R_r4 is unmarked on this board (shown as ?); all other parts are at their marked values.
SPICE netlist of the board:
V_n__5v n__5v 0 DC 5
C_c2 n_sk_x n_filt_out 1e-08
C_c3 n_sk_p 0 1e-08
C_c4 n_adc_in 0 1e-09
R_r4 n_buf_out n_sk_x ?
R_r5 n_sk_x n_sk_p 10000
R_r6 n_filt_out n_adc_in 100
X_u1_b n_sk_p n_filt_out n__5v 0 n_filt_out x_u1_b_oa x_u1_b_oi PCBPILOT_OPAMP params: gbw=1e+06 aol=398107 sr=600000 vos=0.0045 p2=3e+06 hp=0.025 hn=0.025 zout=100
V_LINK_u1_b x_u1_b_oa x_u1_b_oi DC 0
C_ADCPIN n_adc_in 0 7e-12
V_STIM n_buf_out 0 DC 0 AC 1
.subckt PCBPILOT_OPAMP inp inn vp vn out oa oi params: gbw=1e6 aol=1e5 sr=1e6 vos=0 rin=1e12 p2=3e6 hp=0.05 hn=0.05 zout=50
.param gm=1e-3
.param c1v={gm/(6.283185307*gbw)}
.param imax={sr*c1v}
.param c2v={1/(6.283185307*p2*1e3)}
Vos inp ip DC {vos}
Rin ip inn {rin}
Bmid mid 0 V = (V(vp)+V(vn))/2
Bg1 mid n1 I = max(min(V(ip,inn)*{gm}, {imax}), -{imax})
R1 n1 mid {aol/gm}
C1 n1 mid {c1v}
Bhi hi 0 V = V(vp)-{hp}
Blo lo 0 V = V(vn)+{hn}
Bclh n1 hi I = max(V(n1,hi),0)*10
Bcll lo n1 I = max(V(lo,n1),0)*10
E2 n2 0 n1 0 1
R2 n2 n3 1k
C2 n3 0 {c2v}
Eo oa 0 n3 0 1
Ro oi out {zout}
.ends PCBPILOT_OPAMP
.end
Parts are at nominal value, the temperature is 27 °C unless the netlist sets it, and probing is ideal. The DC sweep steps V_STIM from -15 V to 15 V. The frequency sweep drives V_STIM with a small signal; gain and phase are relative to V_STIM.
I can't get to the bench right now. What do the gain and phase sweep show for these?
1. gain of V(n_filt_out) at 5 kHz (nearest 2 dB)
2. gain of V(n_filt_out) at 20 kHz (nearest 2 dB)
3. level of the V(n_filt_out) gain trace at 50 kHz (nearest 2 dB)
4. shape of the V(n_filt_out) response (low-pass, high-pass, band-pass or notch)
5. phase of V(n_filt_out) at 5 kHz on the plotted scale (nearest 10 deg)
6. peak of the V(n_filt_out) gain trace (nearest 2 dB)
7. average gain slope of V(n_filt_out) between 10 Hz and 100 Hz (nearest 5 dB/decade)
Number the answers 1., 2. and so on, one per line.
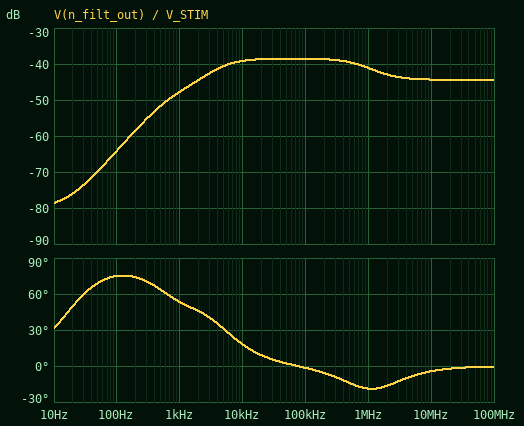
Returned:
1. -40 dB
2. -38 dB
3. -38 dB
4. high-pass
5. 30 deg
6. -38 dB
7. 15 dB/decade
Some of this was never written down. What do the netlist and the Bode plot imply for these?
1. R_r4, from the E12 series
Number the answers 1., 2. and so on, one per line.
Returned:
1. 8.2 kΩ
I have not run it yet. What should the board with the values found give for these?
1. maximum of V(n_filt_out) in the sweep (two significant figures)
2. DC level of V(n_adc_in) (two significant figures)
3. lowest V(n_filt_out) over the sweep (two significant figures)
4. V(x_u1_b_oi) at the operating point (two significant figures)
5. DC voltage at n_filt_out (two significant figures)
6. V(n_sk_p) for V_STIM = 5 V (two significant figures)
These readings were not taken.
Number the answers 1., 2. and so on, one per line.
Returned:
1. 5.0 V
2. 25 mV
3. 25 mV
4. 25 mV
5. 25 mV
6. 5.0 V
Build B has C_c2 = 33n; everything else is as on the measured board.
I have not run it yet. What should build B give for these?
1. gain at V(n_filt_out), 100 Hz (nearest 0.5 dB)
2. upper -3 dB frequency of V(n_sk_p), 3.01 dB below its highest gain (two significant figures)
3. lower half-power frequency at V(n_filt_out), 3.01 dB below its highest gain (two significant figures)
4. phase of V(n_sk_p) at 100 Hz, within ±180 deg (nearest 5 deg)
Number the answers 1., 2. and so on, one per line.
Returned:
1. -54.0 dB
2. 400 Hz
3. 950 Hz
4. -15 deg
